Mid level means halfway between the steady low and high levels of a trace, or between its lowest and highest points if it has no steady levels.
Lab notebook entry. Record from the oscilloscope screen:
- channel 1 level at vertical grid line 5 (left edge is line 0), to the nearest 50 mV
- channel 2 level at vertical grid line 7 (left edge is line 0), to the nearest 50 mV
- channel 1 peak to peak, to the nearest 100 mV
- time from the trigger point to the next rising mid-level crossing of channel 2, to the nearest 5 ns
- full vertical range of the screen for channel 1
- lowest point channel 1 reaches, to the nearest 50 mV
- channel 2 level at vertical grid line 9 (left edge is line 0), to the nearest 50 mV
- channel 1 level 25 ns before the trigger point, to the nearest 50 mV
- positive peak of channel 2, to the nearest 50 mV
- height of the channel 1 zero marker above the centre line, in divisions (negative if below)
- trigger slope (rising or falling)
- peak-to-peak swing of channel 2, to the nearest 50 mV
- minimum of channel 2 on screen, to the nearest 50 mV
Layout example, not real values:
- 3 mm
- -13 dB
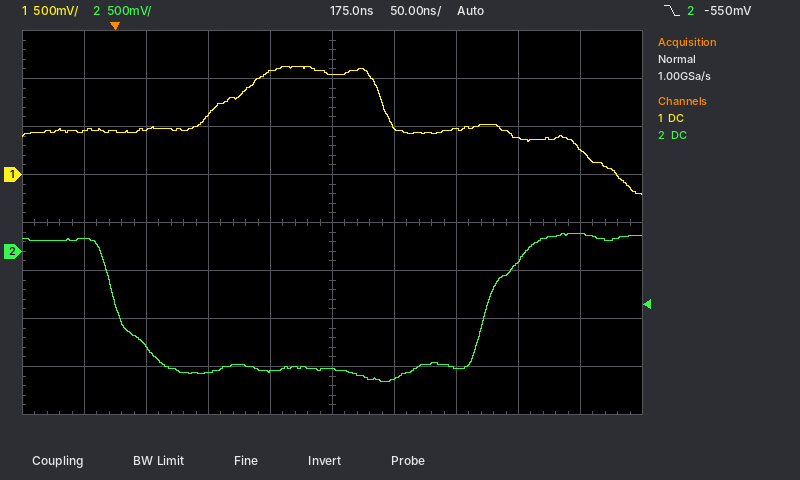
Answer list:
- 1.05 V
- -1.20 V
- 1.30 V
- 300 ns
- 4 V
- -200 mV
- 200 mV
- 450 mV
- 200 mV
- +1.0 div
- falling
- 1.55 V
- -1.35 V
